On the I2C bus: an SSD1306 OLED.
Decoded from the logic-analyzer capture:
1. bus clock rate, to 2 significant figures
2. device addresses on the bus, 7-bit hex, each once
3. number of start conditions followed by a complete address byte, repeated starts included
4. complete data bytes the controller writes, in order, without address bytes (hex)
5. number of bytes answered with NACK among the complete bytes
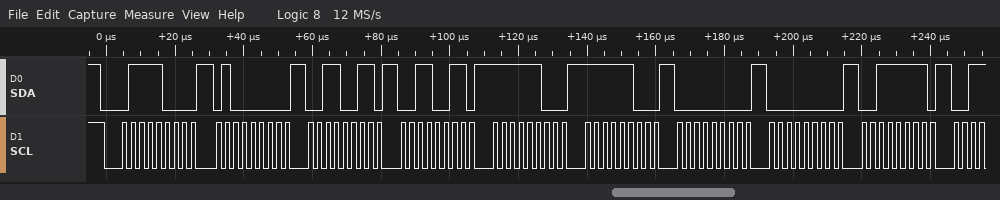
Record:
400 kHz
0x3C
1
40 33 33 FC FC 00 00 3F
0
